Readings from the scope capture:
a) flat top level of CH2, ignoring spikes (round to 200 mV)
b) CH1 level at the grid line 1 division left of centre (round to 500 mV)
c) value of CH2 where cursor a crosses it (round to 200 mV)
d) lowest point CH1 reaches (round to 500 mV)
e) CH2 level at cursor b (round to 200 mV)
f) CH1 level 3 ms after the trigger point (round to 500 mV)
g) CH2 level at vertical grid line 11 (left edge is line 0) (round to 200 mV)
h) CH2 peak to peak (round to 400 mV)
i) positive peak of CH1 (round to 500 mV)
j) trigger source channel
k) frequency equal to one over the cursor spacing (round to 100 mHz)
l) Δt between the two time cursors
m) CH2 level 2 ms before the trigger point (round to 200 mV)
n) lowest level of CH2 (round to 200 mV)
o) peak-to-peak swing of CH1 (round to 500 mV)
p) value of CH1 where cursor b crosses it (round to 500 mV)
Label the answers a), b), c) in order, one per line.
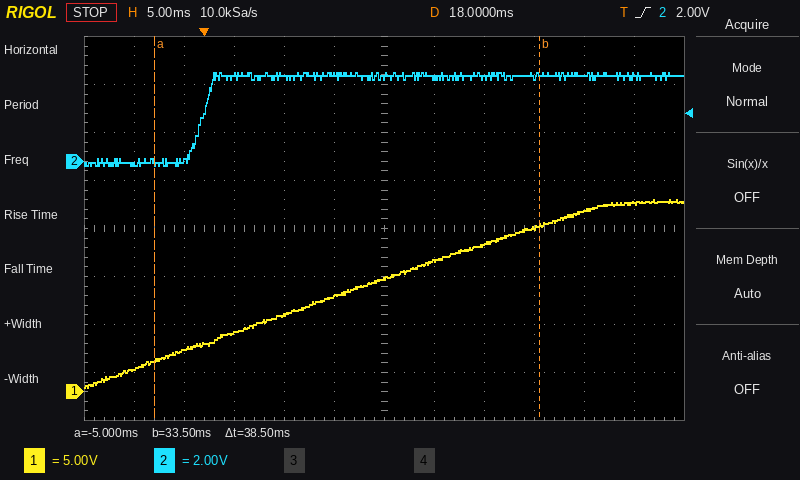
a) 3.6 V
b) 10.0 V
c) 0.0 V
d) 500 mV
e) 3.6 V
f) 6.0 V
g) 3.6 V
h) 4.0 V
i) 20.0 V
j) CH2
k) 26.0 Hz
l) 38.5 ms
m) 0.0 V
n) -200 mV
o) 19.5 V
p) 17.5 V
